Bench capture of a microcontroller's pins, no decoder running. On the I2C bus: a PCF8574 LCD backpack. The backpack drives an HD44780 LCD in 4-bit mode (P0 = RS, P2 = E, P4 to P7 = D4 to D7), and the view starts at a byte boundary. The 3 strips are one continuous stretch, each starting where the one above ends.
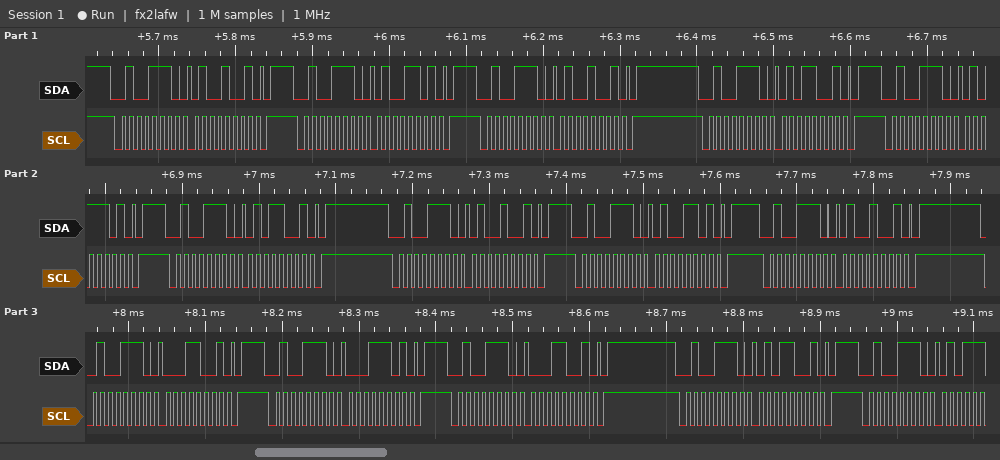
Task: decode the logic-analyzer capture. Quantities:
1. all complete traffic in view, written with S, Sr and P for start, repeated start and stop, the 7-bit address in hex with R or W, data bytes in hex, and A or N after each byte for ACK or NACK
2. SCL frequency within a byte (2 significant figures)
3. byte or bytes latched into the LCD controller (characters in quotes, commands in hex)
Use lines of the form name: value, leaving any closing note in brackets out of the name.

all complete traffic in view, written with S, Sr and P for start, repeated start and stop, the 7-bit address in hex with R or W, data bytes in hex, and A or N after each byte for ACK or NACK: S 27W A 49 A P S 27W A 4D A P S 27W A 49 A P S 27W A 59 A P S 27W A 5D A P S 27W A 59 A P S 27W A 49 A P S 27W A 4D A P S 27W A 49 A P S 27W A 19 A P S 27W A 1D A P S 27W A 19 A P S 27W A 59 A P S 27W A
SCL frequency within a byte: 100 kHz
byte or bytes latched into the LCD controller: 'E' 'A'
